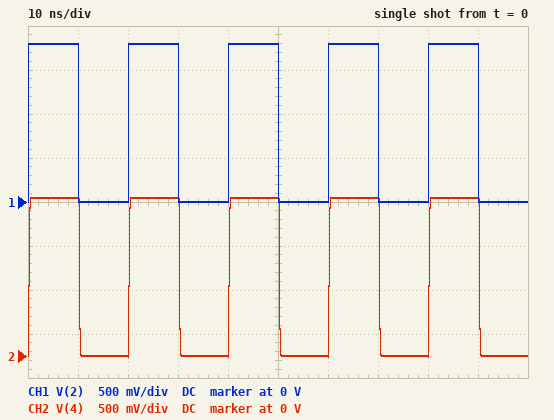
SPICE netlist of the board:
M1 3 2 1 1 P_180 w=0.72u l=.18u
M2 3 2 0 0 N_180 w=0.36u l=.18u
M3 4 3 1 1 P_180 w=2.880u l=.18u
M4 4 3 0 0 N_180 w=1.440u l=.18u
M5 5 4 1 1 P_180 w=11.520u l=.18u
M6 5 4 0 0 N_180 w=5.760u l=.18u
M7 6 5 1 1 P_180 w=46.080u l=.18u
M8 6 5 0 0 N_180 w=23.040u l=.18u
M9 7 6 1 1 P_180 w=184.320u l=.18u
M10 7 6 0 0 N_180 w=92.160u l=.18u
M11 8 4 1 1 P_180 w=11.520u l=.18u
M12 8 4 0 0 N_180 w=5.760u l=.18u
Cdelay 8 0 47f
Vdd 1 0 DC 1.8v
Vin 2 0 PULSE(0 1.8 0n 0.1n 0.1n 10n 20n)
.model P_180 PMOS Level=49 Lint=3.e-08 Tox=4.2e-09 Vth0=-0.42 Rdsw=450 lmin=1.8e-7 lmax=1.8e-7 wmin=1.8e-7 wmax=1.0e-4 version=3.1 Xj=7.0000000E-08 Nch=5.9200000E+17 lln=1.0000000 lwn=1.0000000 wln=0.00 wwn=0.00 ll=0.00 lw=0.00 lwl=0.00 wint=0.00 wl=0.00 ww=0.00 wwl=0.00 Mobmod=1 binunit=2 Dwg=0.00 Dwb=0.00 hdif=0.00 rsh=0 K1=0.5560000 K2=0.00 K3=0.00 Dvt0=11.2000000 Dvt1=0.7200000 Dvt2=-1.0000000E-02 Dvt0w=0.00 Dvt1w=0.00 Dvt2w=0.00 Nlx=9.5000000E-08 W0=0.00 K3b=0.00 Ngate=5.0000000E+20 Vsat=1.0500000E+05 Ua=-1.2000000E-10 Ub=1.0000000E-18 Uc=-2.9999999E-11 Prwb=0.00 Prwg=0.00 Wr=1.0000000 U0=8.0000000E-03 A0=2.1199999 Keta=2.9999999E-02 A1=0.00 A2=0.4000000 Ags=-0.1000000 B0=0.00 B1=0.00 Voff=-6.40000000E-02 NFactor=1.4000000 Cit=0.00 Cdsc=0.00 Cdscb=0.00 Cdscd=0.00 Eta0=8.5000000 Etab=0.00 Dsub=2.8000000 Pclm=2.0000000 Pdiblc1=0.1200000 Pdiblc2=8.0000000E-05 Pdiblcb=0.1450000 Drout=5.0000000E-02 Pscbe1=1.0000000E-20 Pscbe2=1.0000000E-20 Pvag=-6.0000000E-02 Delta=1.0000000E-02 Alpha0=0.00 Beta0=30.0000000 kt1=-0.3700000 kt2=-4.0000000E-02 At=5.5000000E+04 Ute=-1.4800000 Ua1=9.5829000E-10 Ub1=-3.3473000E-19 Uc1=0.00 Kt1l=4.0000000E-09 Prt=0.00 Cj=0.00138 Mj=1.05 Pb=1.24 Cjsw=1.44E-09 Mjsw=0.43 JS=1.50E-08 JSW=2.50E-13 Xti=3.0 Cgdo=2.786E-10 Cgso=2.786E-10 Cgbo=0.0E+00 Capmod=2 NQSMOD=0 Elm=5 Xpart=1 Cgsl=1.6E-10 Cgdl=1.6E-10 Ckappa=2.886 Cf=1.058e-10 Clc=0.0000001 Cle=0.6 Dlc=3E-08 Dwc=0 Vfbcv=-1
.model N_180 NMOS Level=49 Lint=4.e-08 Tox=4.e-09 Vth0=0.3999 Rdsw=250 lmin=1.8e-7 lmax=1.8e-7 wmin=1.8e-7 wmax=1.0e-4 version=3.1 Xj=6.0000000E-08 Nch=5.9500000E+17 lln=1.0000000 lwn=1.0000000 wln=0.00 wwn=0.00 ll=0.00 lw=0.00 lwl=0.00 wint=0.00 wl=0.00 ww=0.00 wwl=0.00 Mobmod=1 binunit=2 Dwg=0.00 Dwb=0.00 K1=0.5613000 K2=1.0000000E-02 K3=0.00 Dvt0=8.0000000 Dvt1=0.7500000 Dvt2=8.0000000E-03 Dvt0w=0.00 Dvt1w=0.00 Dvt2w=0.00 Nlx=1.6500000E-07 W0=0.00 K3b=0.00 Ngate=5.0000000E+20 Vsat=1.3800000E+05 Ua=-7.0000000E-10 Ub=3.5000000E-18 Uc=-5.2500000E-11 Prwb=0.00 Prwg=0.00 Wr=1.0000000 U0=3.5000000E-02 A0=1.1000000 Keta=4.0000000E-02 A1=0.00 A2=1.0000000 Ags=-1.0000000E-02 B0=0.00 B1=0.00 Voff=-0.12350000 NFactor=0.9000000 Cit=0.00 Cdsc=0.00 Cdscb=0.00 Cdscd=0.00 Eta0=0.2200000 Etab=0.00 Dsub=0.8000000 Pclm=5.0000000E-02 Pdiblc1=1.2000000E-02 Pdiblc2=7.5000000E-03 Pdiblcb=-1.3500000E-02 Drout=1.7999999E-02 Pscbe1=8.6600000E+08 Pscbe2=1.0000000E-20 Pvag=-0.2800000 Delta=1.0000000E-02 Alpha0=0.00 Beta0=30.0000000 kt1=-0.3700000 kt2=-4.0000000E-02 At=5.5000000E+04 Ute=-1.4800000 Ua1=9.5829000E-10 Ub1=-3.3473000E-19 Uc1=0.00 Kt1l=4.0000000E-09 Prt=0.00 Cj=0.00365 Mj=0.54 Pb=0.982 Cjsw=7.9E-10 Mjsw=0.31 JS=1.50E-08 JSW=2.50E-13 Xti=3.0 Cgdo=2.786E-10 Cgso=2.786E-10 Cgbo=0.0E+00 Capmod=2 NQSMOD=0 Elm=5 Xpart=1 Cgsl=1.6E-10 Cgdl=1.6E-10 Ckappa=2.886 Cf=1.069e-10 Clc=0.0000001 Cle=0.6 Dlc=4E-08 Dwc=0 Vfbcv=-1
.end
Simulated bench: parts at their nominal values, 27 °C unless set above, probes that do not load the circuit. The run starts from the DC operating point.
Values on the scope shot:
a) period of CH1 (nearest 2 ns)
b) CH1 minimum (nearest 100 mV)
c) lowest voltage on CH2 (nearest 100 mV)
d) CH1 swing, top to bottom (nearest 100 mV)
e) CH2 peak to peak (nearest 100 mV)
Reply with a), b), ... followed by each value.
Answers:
a) 20 ns
b) 0 V
c) 0 V
d) 1.8 V
e) 1.8 V
